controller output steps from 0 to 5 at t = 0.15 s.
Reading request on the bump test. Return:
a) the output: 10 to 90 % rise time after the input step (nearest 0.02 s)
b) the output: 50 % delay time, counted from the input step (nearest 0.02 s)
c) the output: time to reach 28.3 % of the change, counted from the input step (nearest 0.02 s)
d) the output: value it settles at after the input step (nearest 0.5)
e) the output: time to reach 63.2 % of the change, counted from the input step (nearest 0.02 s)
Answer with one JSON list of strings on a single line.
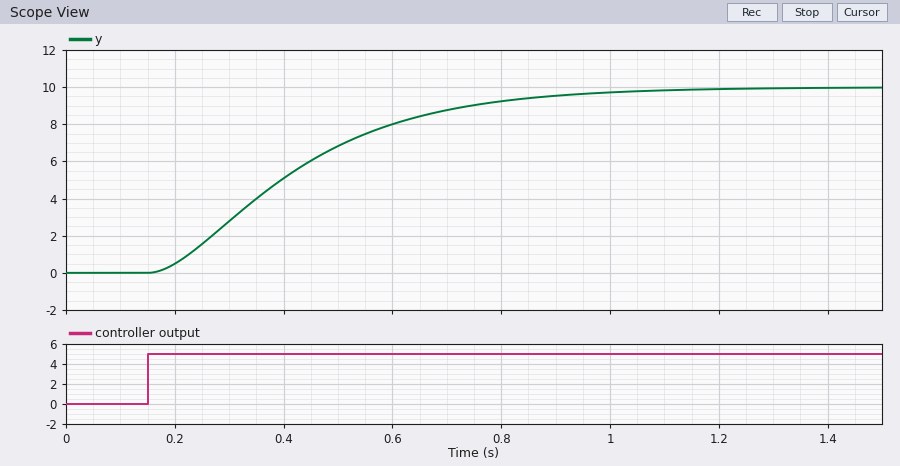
["0.52 s", "0.24 s", "0.16 s", "10.0", "0.32 s"]
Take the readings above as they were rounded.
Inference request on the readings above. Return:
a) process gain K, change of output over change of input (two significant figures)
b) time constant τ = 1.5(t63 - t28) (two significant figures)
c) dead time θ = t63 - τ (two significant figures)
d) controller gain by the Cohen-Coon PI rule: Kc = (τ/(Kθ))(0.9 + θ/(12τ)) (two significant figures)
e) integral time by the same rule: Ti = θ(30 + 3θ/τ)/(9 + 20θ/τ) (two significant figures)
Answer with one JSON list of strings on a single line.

["2.0", "0.24 s", "0.080 s", "1.4", "0.16 s"]
